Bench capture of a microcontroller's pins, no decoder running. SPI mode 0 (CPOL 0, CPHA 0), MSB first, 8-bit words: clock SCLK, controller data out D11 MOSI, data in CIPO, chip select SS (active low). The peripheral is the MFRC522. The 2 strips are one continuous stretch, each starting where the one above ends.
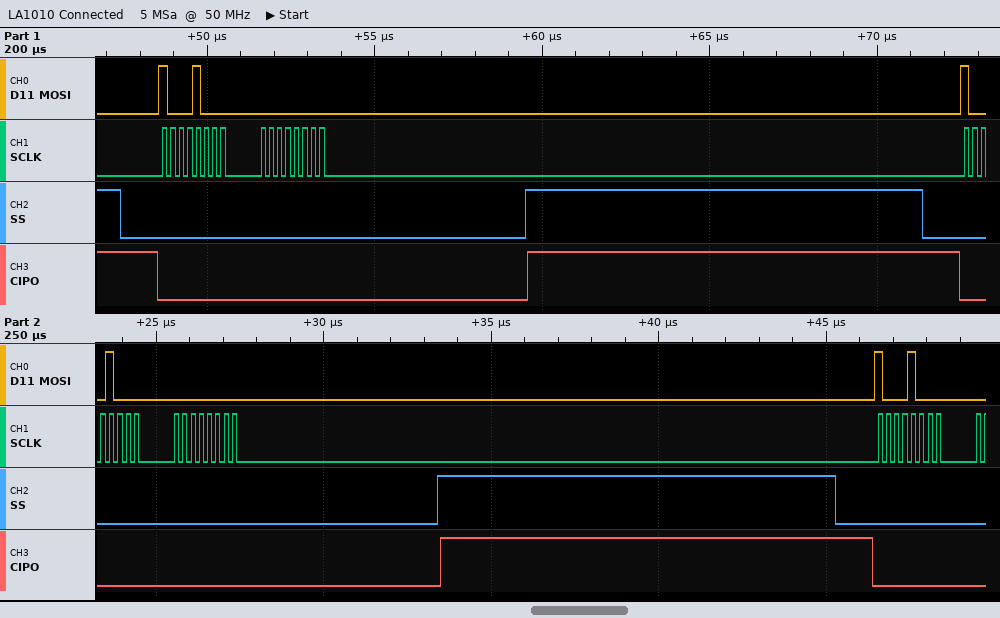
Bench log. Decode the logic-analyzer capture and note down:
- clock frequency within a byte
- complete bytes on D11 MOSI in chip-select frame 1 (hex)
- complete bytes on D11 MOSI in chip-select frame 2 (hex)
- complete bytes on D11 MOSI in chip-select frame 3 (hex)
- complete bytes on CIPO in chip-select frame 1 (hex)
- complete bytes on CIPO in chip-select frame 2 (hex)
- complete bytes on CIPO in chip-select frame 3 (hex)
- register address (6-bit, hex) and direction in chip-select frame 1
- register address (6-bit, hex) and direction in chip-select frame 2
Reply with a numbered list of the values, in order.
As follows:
1. 4 MHz
2. 0x88 0x00
3. 0x88 0x00
4. 0x88
5. 0x00 0x00
6. 0x00 0x00
7. 0x00
8. 0x04 read
9. 0x04 read
